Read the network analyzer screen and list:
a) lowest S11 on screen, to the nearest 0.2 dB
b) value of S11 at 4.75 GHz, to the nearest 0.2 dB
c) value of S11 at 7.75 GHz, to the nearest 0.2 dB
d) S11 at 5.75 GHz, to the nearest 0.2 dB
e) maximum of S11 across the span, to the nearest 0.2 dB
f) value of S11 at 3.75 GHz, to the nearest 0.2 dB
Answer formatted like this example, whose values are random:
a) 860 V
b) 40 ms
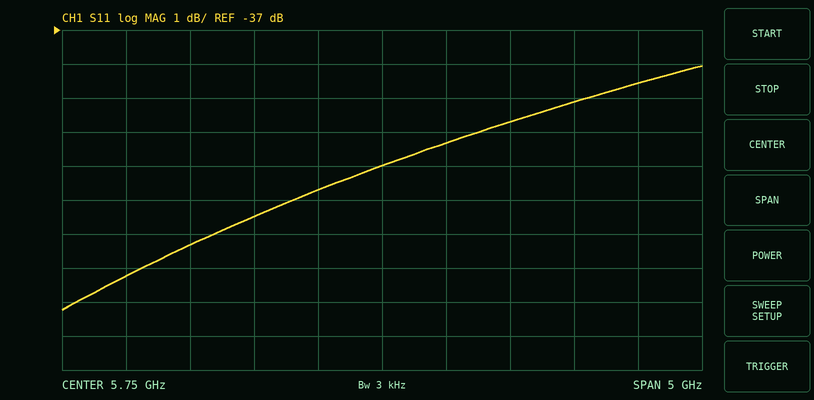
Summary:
a) -45.2 dB
b) -42.4 dB
c) -38.6 dB
d) -41.0 dB
e) -38.0 dB
f) -44.2 dB
